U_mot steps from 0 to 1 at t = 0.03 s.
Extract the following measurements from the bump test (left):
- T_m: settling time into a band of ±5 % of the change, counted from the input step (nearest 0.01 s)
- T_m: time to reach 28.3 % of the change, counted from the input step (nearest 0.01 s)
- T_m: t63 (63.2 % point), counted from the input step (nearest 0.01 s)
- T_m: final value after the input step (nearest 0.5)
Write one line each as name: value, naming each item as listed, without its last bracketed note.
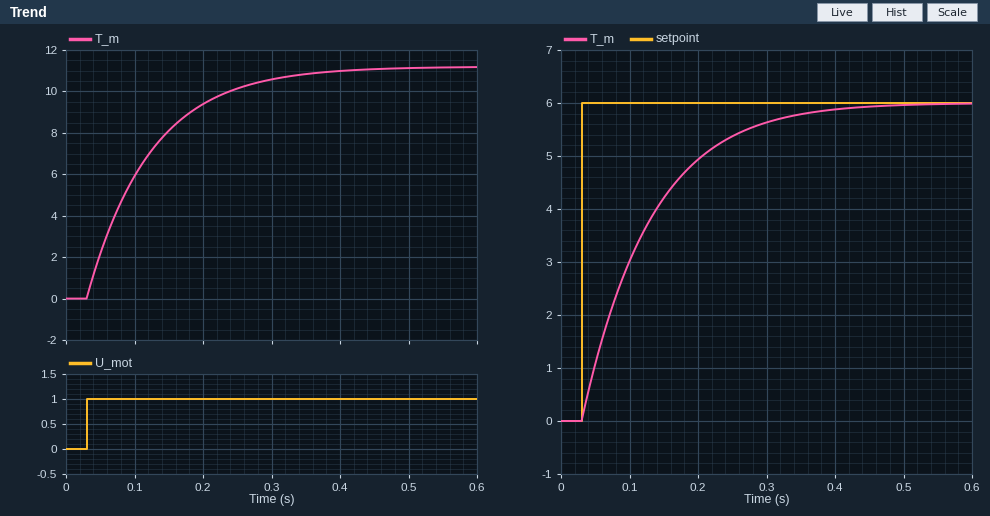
T_m: settling time into a band of ±5 % of the change, counted from the input step: 0.28 s
T_m: time to reach 28.3 % of the change, counted from the input step: 0.03 s
T_m: t63 (63.2 % point), counted from the input step: 0.09 s
T_m: final value after the input step: 11.0
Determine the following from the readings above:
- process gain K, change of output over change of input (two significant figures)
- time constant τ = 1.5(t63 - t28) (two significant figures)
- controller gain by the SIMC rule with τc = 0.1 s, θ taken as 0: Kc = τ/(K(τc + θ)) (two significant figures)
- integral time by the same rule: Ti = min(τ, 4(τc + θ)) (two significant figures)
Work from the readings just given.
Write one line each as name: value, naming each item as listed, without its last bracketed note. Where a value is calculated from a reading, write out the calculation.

process gain K, change of output over change of input: (11 - 0) / 1 = 11
time constant τ = 1.5(t63 - t28): 1.5 × (0.09 - 0.03) = 0.090 s
controller gain by the SIMC rule with τc = 0.1 s, θ taken as 0: Kc = τ/(K(τc + θ)): 0.09 / (11 × (0.1 + 0)) = 0.082
integral time by the same rule: Ti = min(τ, 4(τc + θ)): min(0.09, 4 × (0.1 + 0)) = 0.090 s
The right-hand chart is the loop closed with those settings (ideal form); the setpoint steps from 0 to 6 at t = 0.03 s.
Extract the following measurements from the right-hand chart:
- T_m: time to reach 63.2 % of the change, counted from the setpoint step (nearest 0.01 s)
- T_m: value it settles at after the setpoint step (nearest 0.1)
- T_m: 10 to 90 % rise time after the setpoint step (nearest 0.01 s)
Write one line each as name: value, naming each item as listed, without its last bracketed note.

T_m: time to reach 63.2 % of the change, counted from the setpoint step: 0.10 s
T_m: value it settles at after the setpoint step: 6.0
T_m: 10 to 90 % rise time after the setpoint step: 0.21 s
